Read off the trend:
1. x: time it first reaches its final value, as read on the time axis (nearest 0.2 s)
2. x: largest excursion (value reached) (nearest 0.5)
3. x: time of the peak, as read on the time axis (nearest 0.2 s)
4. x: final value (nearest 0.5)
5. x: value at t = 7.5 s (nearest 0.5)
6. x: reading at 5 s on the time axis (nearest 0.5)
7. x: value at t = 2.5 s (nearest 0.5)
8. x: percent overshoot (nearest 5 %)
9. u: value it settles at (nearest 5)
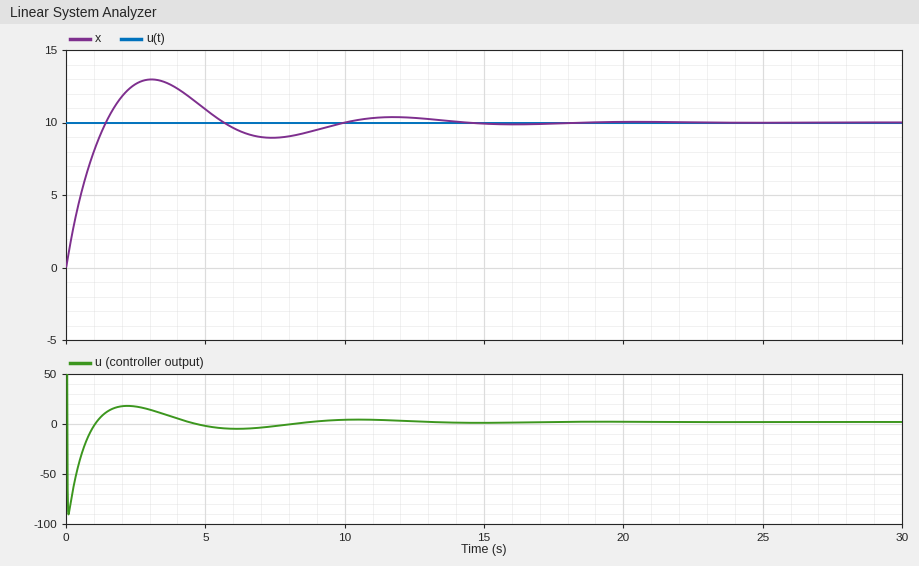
1.4 s
13.0
3.0 s
10.0
9.0
11.0
12.5
30 %
0
